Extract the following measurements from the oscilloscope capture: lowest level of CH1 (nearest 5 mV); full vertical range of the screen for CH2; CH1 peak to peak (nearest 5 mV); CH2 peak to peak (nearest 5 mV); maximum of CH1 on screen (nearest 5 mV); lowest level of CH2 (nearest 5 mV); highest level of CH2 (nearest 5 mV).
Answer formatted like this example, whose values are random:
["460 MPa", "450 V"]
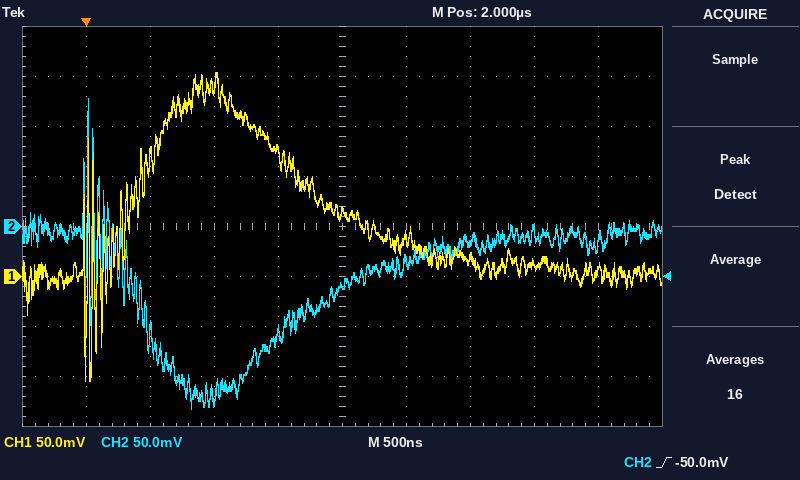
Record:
["-105 mV", "400 mV", "310 mV", "310 mV", "205 mV", "-180 mV", "130 mV"]
